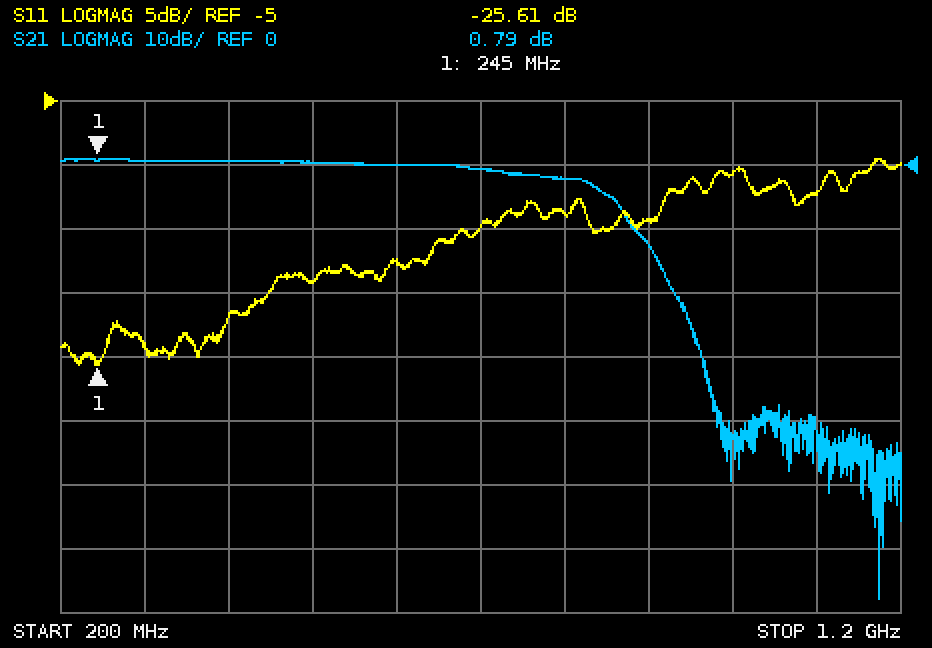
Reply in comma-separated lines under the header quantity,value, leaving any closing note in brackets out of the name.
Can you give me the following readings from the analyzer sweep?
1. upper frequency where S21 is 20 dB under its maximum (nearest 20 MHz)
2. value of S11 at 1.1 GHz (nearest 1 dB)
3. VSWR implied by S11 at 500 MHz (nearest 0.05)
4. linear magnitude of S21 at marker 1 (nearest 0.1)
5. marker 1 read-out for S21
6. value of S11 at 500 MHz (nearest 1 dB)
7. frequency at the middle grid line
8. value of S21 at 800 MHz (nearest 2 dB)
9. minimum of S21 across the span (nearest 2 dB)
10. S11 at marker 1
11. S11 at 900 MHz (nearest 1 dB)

quantity,value
upper frequency where S21 is 20 dB under its maximum,920 MHz
value of S11 at 1.1 GHz,-12 dB
VSWR implied by S11 at 500 MHz,1.25
linear magnitude of S21 at marker 1,1.1
marker 1 read-out for S21,0.79 dB
value of S11 at 500 MHz,-19 dB
frequency at the middle grid line,700 MHz
value of S21 at 800 MHz,-2 dB
minimum of S21 across the span,-68 dB
S11 at marker 1,-25.61 dB
S11 at 900 MHz,-14 dB
